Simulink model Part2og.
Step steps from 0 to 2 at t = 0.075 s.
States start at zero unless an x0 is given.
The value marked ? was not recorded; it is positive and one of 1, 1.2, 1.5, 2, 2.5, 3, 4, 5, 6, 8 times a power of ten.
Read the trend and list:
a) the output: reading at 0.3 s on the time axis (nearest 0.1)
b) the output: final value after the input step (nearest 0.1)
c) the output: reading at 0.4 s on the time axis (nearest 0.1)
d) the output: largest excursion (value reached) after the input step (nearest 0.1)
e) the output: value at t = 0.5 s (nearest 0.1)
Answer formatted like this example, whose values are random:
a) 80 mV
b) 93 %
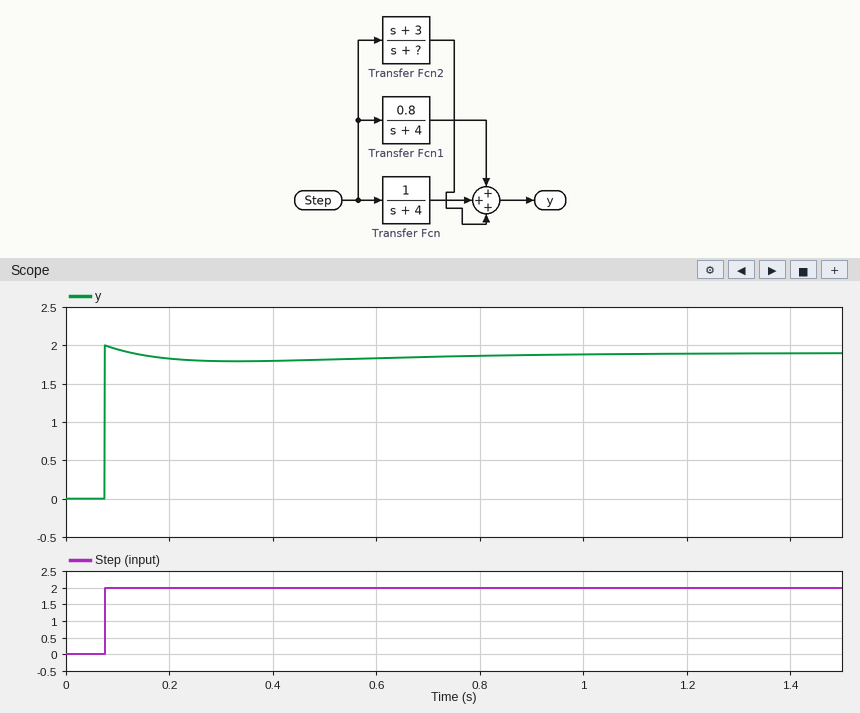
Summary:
a) 1.8
b) 1.9
c) 1.8
d) 2.0
e) 1.8
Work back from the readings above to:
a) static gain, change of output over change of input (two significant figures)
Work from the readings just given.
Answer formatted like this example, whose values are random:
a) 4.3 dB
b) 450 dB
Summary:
a) 0.95
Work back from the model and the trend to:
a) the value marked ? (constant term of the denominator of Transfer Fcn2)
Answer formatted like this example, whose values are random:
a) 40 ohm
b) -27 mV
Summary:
a) 6
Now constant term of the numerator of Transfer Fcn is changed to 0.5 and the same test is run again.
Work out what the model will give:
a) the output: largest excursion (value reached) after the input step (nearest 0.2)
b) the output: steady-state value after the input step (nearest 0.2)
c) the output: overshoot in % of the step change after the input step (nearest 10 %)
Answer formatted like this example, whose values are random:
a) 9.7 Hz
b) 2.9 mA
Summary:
a) 2.0
b) 1.6
c) 20 %
